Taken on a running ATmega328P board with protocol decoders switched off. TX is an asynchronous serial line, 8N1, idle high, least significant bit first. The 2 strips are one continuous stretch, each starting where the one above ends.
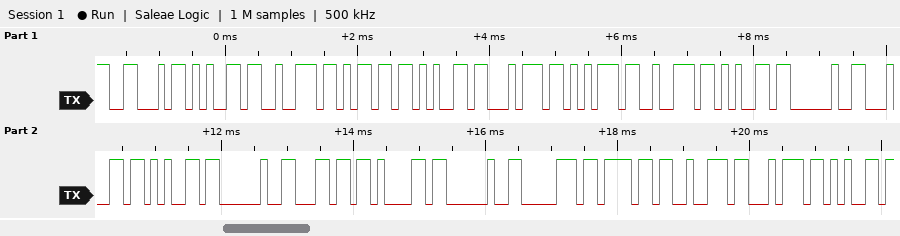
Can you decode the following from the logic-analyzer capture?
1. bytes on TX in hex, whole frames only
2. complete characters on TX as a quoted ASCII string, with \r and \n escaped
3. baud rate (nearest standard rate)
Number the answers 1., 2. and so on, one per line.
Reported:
1. 46 65 72 6D 65 74 75 72 65 20 64 65 20 6C 61 20 70 6F 72 74 65
2. "Fermeture de la porte"
3. 9600 baud
